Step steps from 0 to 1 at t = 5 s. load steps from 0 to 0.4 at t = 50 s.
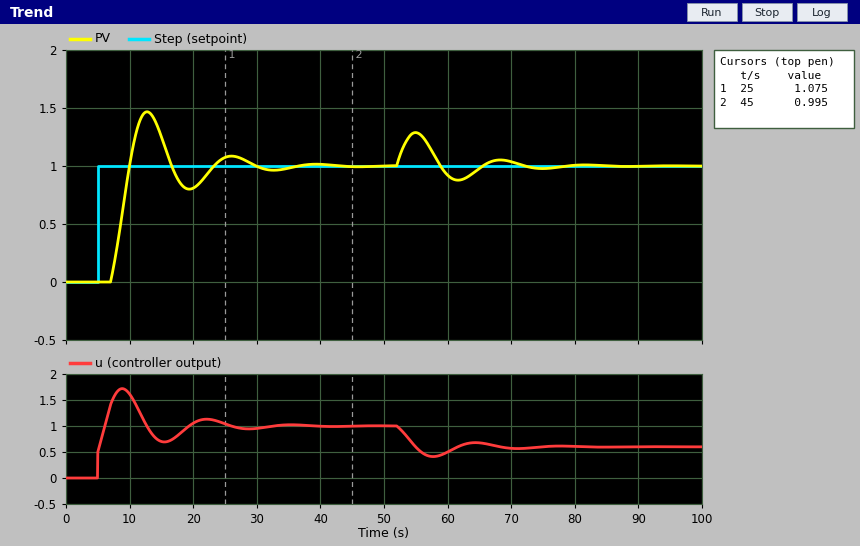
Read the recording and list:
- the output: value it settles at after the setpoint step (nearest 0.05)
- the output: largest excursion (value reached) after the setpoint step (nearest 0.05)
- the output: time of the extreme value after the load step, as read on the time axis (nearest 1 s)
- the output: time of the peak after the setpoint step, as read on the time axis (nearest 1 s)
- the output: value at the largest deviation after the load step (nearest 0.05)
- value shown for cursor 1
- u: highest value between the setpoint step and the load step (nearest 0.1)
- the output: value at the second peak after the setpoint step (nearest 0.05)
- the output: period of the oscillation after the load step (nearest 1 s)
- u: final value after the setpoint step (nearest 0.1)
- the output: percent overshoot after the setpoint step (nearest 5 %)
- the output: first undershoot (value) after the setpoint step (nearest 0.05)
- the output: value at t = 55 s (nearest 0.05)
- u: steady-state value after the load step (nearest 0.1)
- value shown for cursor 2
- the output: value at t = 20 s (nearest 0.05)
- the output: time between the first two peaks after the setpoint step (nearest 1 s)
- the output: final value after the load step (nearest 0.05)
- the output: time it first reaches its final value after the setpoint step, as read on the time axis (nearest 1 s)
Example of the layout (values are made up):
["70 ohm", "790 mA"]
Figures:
["1.00", "1.45", "55 s", "13 s", "1.30", "1.075", "1.7", "1.10", "13 s", "1.0", "45 %", "0.80", "1.30", "0.6", "0.995", "0.80", "13 s", "1.00", "10 s"]
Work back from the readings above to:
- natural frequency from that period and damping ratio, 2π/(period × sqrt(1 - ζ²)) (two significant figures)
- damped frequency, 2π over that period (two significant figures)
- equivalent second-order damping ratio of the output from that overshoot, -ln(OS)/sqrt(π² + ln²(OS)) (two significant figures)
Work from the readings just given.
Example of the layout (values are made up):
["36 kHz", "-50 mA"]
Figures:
["0.50 rad/s", "0.48 rad/s", "0.25"]
